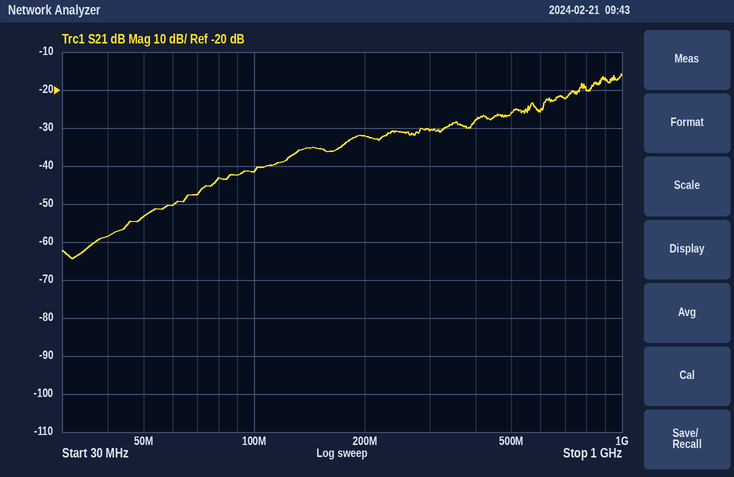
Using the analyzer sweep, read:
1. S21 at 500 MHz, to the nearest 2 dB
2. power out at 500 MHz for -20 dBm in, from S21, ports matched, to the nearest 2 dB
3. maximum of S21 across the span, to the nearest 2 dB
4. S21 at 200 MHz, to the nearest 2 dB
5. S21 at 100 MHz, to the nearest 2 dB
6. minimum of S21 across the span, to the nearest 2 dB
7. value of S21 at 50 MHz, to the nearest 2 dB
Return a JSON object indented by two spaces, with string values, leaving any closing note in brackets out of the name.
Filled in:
{
  "S21 at 500 MHz, to the nearest 2 dB": "-26 dB",
  "power out at 500 MHz for -20 dBm in, from S21, ports matched, to the nearest 2 dB": "-46 dBm",
  "maximum of S21 across the span, to the nearest 2 dB": "-16 dB",
  "S21 at 200 MHz, to the nearest 2 dB": "-32 dB",
  "S21 at 100 MHz, to the nearest 2 dB": "-42 dB",
  "minimum of S21 across the span, to the nearest 2 dB": "-64 dB",
  "value of S21 at 50 MHz, to the nearest 2 dB": "-54 dB"
}
